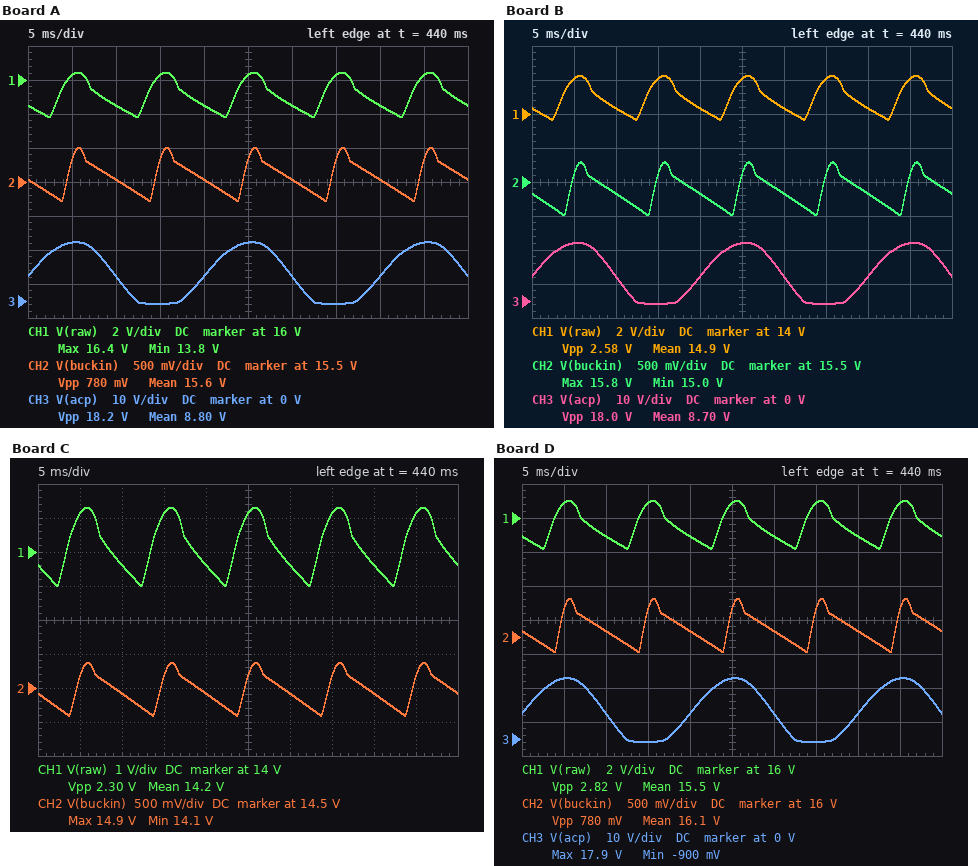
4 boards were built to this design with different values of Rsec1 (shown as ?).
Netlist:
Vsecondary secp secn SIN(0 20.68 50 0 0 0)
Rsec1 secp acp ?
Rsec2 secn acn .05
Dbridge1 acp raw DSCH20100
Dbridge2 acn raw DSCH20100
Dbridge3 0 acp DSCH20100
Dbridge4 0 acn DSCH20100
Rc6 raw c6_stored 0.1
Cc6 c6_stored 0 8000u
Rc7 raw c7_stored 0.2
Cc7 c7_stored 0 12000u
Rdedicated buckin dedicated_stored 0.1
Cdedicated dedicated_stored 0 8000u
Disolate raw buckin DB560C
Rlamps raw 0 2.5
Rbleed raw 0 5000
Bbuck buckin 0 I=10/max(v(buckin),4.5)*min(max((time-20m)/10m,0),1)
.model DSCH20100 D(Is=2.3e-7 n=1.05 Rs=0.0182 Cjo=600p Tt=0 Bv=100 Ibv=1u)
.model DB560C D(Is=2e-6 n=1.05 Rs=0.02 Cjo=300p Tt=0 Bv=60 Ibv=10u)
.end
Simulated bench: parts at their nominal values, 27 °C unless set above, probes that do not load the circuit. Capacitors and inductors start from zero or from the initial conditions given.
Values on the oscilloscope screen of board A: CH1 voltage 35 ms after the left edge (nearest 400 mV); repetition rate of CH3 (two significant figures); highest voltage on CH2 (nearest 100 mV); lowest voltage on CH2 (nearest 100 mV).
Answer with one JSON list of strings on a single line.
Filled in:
["16.4 V", "50 Hz", "16.0 V", "15.2 V"]
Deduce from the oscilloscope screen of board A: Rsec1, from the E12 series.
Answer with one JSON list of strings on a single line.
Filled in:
["0.068 Ω"]
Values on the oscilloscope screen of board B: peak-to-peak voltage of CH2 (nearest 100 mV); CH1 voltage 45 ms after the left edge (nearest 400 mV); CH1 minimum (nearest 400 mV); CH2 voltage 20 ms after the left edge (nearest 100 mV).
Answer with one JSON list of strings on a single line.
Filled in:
["800 mV", "16.0 V", "13.6 V", "15.3 V"]
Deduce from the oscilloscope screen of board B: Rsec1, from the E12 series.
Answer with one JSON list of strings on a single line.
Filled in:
["0.082 Ω"]
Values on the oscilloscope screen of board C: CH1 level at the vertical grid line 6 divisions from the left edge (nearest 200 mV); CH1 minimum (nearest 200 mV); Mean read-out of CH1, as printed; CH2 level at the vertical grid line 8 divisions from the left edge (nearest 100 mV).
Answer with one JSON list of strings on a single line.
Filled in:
["13.6 V", "13.0 V", "14.2 V", "14.4 V"]
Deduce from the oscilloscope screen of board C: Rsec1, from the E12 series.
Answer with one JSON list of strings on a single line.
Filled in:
["0.15 Ω"]
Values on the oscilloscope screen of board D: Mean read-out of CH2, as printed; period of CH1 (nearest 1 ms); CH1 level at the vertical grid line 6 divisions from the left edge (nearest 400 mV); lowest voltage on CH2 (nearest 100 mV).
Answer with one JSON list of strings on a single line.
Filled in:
["16.1 V", "10 ms", "14.8 V", "15.8 V"]
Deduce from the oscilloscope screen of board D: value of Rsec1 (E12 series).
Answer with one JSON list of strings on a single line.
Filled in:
["0.033 Ω"]
